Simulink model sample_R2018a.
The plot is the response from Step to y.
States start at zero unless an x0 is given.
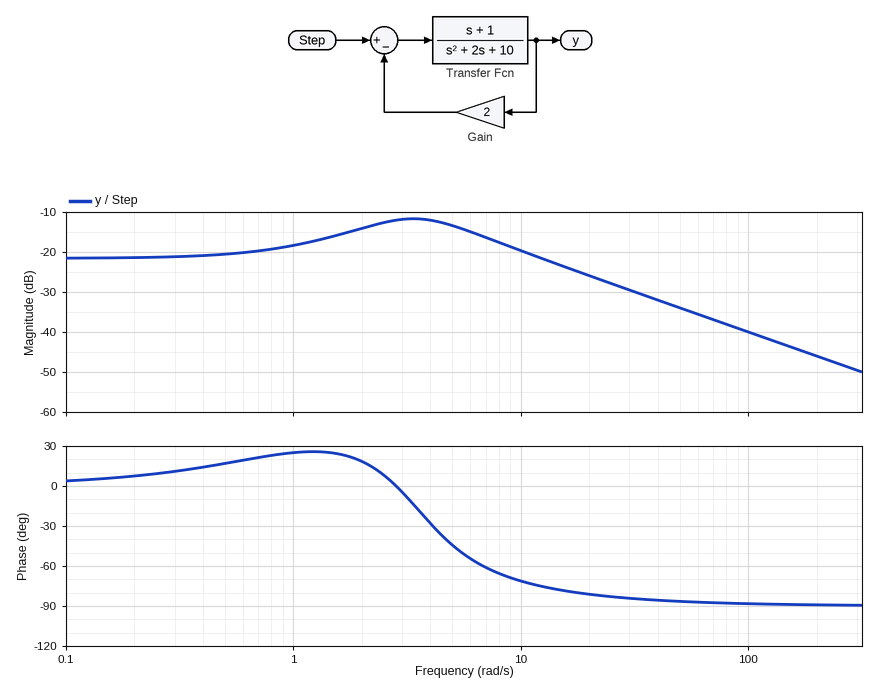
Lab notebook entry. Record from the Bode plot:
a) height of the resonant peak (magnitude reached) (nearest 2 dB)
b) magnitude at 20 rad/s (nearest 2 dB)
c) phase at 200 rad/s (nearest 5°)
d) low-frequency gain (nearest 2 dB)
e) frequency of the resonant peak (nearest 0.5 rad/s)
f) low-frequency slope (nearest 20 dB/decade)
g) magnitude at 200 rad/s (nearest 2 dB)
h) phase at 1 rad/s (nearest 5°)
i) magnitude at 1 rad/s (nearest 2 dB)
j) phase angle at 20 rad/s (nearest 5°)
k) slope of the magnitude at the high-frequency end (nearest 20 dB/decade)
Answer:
-12 dB
-26 dB
-90°
-22 dB
3.5 rad/s
0 dB/decade
-46 dB
25°
-18 dB
-80°
-20 dB/decade
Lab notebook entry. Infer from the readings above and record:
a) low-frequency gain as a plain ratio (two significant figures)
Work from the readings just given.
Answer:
0.079
